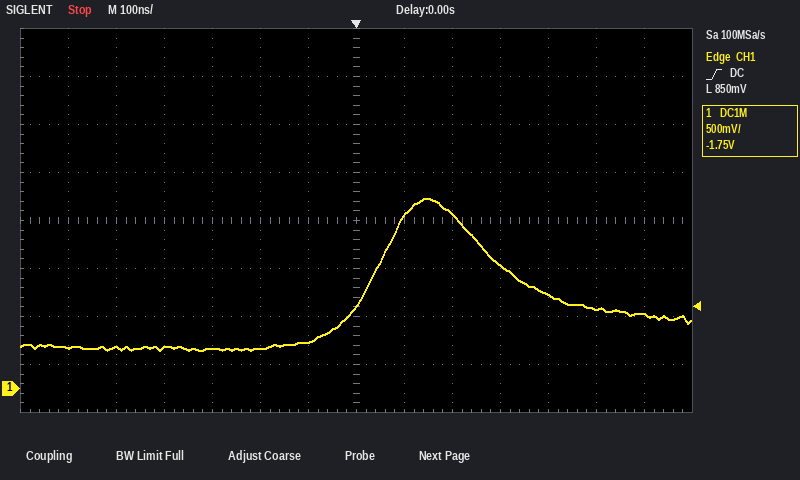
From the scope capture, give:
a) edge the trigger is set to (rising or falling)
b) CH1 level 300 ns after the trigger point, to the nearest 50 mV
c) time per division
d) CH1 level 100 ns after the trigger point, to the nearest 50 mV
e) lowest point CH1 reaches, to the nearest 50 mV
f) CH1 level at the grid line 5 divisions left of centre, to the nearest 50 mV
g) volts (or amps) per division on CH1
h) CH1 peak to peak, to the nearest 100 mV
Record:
rising
1.30 V
100 ns
1.80 V
400 mV
450 mV
500 mV
1.60 V
